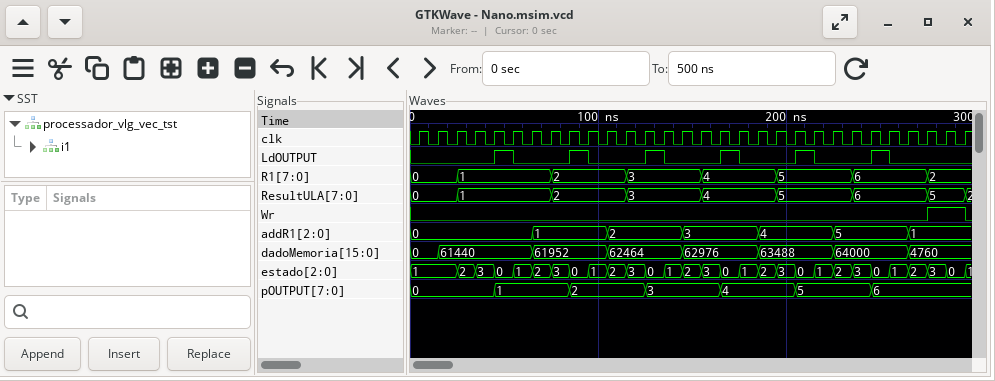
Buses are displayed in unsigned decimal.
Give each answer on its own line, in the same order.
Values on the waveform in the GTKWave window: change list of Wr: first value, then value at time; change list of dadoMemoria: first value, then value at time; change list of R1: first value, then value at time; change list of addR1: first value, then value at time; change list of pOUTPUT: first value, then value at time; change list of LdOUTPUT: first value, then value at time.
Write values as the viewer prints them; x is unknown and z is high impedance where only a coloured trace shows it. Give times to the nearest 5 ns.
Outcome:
0, 1 at 275 ns, 0 at 295 ns
0, 61440 at 15 ns, 61952 at 65 ns, 62464 at 105 ns, 62976 at 145 ns, 63488 at 185 ns, 64000 at 225 ns, 4760 at 265 ns
0, 1 at 25 ns, 2 at 75 ns, 3 at 115 ns, 4 at 155 ns, 5 at 195 ns, 6 at 235 ns, 2 at 275 ns
0, 1 at 65 ns, 2 at 105 ns, 3 at 145 ns, 4 at 185 ns, 5 at 225 ns, 1 at 265 ns
0, 1 at 45 ns, 2 at 85 ns, 3 at 125 ns, 4 at 165 ns, 5 at 205 ns, 6 at 245 ns
0, 1 at 45 ns, 0 at 55 ns, 1 at 85 ns, 0 at 95 ns, 1 at 125 ns, 0 at 135 ns, 1 at 165 ns, 0 at 175 ns, 1 at 205 ns, 0 at 215 ns, 1 at 245 ns, 0 at 255 ns
